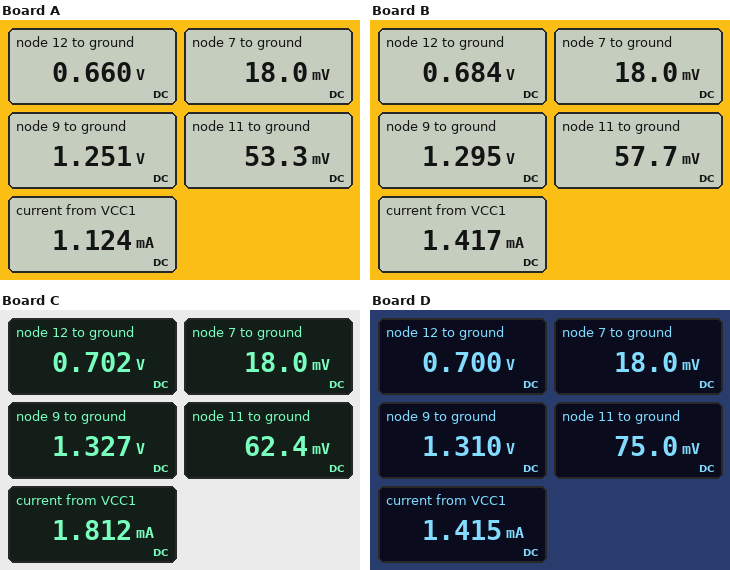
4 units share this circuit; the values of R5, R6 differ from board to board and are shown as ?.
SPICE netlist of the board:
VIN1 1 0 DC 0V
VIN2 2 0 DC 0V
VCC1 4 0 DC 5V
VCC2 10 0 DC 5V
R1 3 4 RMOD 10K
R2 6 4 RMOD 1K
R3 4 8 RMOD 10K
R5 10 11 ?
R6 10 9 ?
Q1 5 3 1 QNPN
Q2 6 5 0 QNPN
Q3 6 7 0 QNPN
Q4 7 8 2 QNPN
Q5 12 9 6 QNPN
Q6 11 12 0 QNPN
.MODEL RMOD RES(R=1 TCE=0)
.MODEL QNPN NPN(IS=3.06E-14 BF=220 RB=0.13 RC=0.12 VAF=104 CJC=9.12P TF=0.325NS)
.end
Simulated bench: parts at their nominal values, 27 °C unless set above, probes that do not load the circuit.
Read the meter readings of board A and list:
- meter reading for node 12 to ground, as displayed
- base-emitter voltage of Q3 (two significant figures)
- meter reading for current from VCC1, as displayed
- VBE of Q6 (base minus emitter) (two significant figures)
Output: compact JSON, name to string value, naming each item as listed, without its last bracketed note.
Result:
{"meter reading for node 12 to ground, as displayed": "0.660 V", "base-emitter voltage of Q3": "18 mV", "meter reading for current from VCC1, as displayed": "1.124 mA", "VBE of Q6 (base minus emitter)": "660 mV"}
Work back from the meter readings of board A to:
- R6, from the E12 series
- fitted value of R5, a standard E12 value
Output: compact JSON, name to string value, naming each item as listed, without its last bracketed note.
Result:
{"R6, from the E12 series": "15 kΩ", "fitted value of R5, a standard E12 value": "1.8 kΩ"}
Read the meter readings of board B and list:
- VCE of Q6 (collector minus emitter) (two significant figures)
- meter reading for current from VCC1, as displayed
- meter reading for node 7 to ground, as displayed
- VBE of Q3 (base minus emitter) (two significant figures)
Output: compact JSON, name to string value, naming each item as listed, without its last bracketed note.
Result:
{"VCE of Q6 (collector minus emitter)": "58 mV", "meter reading for current from VCC1, as displayed": "1.417 mA", "meter reading for node 7 to ground, as displayed": "18.0 mV", "VBE of Q3 (base minus emitter)": "18 mV"}
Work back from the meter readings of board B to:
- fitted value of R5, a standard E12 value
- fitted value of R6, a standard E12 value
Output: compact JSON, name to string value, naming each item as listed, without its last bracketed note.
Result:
{"fitted value of R5, a standard E12 value": "680 Ω", "fitted value of R6, a standard E12 value": "6.8 kΩ"}
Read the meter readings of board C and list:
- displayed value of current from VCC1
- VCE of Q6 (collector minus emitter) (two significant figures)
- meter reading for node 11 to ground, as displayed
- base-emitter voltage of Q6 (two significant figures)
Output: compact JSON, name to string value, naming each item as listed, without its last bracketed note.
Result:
{"displayed value of current from VCC1": "1.812 mA", "VCE of Q6 (collector minus emitter)": "62 mV", "meter reading for node 11 to ground, as displayed": "62.4 mV", "base-emitter voltage of Q6": "700 mV"}
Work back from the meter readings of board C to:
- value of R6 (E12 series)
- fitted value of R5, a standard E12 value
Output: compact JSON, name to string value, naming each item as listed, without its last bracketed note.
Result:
{"value of R6": "3.9 kΩ", "fitted value of R5, a standard E12 value": "330 Ω"}
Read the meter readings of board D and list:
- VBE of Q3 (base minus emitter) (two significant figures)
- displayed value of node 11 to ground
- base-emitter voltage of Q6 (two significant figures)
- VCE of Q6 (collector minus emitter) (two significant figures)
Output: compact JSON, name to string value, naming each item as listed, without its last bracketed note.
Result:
{"VBE of Q3 (base minus emitter)": "18 mV", "displayed value of node 11 to ground": "75.0 mV", "base-emitter voltage of Q6": "700 mV", "VCE of Q6 (collector minus emitter)": "75 mV"}
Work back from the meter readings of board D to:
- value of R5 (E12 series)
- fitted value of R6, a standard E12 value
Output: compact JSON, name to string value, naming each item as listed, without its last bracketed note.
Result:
{"value of R5": "330 Ω", "fitted value of R6, a standard E12 value": "6.8 kΩ"}
